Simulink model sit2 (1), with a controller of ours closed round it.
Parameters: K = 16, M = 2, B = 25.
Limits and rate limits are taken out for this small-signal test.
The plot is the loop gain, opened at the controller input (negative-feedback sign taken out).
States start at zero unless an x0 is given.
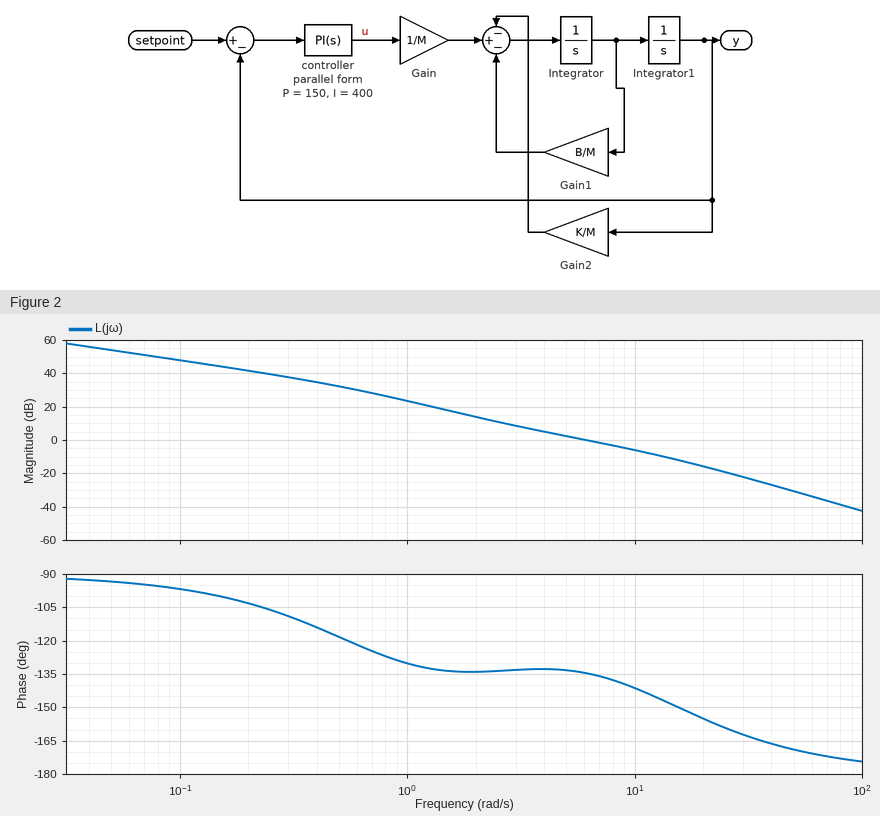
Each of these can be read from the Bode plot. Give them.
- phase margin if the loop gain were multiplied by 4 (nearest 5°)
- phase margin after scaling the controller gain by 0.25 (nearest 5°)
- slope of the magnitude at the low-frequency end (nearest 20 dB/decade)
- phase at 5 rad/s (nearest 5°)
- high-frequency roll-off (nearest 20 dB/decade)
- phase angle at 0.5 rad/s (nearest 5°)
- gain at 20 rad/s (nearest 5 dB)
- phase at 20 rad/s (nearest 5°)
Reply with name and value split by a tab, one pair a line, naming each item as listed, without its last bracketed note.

phase margin if the loop gain were multiplied by 4	30°
phase margin after scaling the controller gain by 0.25	45°
slope of the magnitude at the low-frequency end	-20 dB/decade
phase at 5 rad/s	-135°
high-frequency roll-off	-40 dB/decade
phase angle at 0.5 rad/s	-120°
gain at 20 rad/s	-15 dB
phase at 20 rad/s	-155°
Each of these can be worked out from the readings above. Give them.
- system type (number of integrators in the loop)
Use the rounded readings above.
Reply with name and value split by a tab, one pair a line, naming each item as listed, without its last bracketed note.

system type	1
